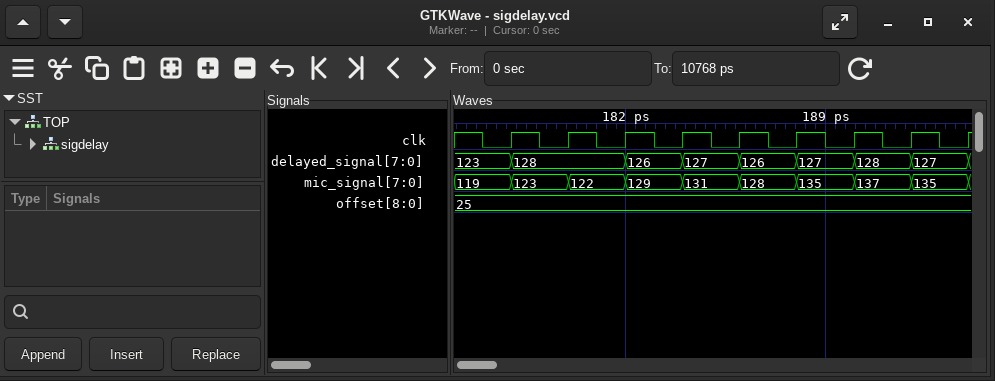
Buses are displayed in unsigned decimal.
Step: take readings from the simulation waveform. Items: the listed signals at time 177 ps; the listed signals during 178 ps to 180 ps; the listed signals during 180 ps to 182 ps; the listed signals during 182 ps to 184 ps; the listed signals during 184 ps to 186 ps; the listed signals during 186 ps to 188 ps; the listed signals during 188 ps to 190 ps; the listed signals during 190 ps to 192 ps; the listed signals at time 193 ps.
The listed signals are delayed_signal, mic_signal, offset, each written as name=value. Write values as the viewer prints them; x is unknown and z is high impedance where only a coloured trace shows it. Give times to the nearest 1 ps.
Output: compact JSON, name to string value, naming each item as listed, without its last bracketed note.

{"the listed signals at time 177 ps": "delayed_signal=123, mic_signal=119, offset=25", "the listed signals during 178 ps to 180 ps": "delayed_signal=128, mic_signal=123, offset=25", "the listed signals during 180 ps to 182 ps": "delayed_signal=128, mic_signal=122, offset=25", "the listed signals during 182 ps to 184 ps": "delayed_signal=126, mic_signal=129, offset=25", "the listed signals during 184 ps to 186 ps": "delayed_signal=127, mic_signal=131, offset=25", "the listed signals during 186 ps to 188 ps": "delayed_signal=126, mic_signal=128, offset=25", "the listed signals during 188 ps to 190 ps": "delayed_signal=127, mic_signal=135, offset=25", "the listed signals during 190 ps to 192 ps": "delayed_signal=128, mic_signal=137, offset=25", "the listed signals at time 193 ps": "delayed_signal=127, mic_signal=135, offset=25"}
